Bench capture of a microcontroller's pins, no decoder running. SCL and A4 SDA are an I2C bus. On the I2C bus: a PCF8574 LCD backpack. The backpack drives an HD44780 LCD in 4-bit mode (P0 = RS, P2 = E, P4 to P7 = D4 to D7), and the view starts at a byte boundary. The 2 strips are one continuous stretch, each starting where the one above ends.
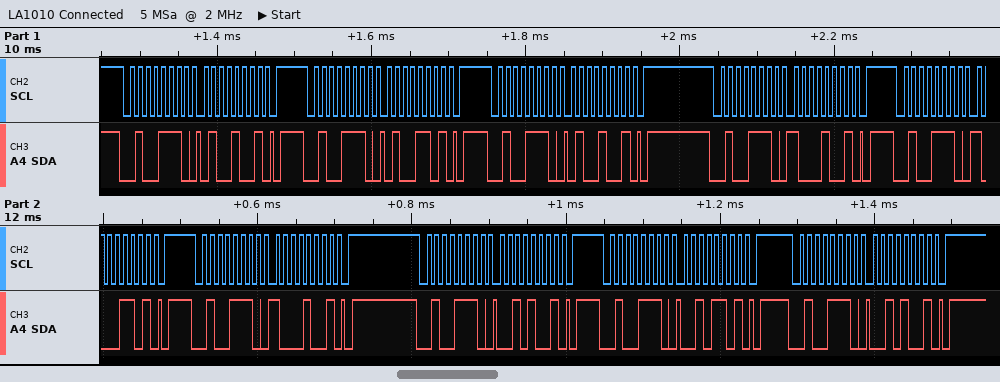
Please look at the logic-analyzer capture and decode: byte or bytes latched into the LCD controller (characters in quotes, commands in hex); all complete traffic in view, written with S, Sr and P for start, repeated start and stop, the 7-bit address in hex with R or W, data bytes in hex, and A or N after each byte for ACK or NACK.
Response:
'H'
S 27W A 49 A P S 27W A 4D A P S 27W A 49 A P S 27W A 89 A P S 27W A 8D A P S 27W A 89 A P S 27W A 29 A P S 27W A 2D A P S 27W A 29 A P
